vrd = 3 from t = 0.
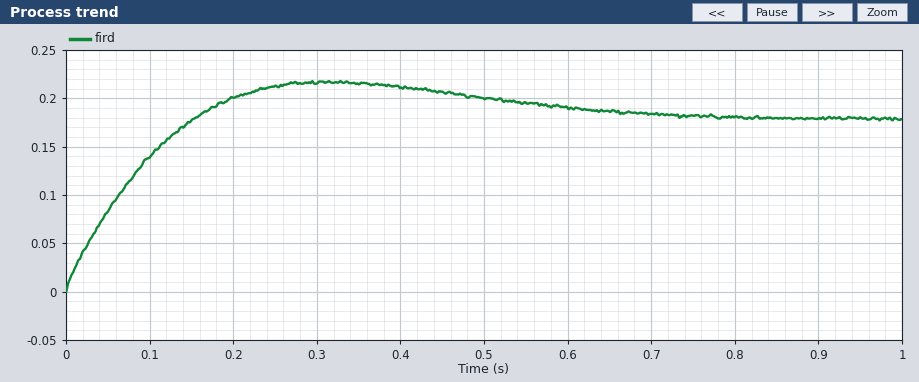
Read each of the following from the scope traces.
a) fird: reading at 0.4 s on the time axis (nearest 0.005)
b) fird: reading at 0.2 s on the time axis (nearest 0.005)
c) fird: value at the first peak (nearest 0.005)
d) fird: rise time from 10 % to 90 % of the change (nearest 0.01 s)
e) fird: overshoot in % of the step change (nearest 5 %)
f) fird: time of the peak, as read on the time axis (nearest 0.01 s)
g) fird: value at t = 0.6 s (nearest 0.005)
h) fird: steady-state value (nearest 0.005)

0.210
0.200
0.215
0.12 s
20 %
0.31 s
0.190
0.180
